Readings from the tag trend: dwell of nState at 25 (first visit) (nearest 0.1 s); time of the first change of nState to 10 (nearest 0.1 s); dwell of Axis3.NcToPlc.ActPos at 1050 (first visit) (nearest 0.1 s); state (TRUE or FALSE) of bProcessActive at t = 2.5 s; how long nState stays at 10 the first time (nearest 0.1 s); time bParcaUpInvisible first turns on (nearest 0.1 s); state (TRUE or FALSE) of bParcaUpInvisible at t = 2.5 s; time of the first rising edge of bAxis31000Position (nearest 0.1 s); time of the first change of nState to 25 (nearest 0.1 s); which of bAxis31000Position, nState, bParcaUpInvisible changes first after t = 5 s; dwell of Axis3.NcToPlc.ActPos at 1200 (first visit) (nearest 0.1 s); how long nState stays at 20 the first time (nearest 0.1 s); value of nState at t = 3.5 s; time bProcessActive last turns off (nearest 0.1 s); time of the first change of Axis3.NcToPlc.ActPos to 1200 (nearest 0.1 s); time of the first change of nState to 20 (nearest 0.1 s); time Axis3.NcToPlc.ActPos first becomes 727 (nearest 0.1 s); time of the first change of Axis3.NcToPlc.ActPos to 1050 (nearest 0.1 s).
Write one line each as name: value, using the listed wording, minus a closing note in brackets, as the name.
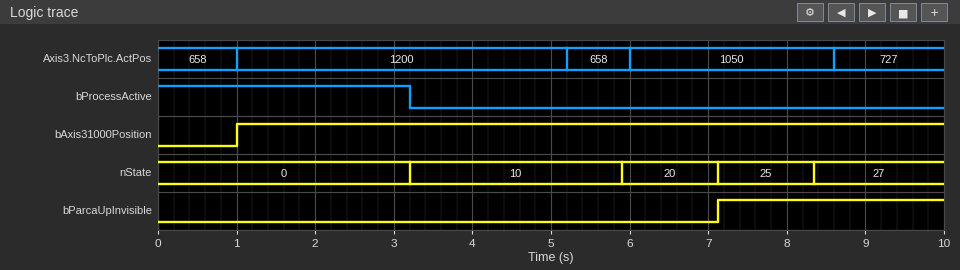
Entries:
dwell of nState at 25 (first visit): 1.2 s
time of the first change of nState to 10: 3.2 s
dwell of Axis3.NcToPlc.ActPos at 1050 (first visit): 2.6 s
state (TRUE or FALSE) of bProcessActive at t = 2.5 s: TRUE
how long nState stays at 10 the first time: 2.7 s
time bParcaUpInvisible first turns on: 7.1 s
state (TRUE or FALSE) of bParcaUpInvisible at t = 2.5 s: FALSE
time of the first rising edge of bAxis31000Position: 1.0 s
time of the first change of nState to 25: 7.1 s
which of bAxis31000Position, nState, bParcaUpInvisible changes first after t = 5 s: nState
dwell of Axis3.NcToPlc.ActPos at 1200 (first visit): 4.2 s
how long nState stays at 20 the first time: 1.2 s
value of nState at t = 3.5 s: 10
time bProcessActive last turns off: 3.2 s
time of the first change of Axis3.NcToPlc.ActPos to 1200: 1.0 s
time of the first change of nState to 20: 5.9 s
time Axis3.NcToPlc.ActPos first becomes 727: 8.6 s
time of the first change of Axis3.NcToPlc.ActPos to 1050: 6.0 s
